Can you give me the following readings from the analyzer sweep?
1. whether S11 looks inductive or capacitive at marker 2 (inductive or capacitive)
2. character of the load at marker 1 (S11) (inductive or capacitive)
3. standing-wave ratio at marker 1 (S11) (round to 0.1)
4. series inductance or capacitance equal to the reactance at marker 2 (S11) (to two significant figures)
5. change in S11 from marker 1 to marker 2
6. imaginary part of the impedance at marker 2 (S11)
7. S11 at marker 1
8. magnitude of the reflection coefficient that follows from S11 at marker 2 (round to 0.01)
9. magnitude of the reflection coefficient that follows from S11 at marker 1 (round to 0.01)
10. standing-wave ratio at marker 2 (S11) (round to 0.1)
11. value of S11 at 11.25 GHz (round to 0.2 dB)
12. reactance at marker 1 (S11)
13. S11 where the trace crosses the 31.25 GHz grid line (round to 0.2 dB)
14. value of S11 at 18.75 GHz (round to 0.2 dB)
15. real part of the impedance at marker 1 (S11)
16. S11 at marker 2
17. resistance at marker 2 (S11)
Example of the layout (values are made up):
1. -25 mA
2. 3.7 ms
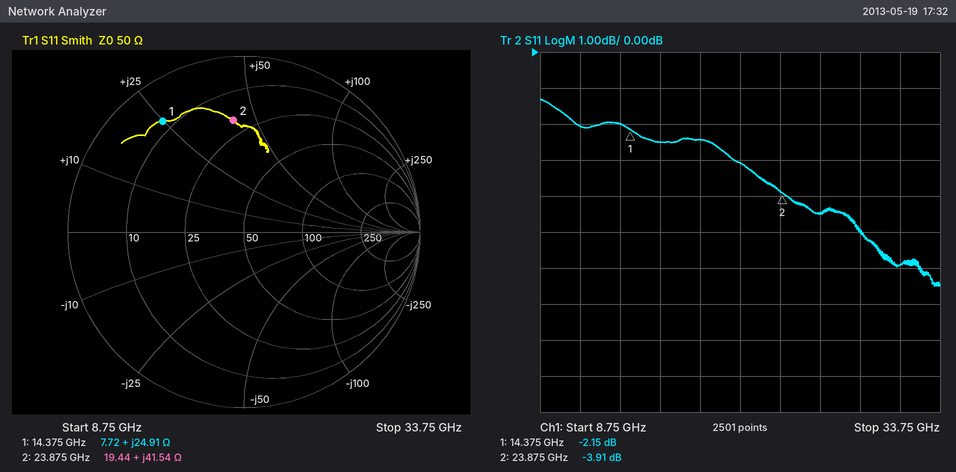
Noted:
1. inductive
2. inductive
3. 8.1
4. 280 pH
5. -1.76 dB
6. +41.54 Ω
7. -2.15 dB
8. 0.64
9. 0.78
10. 4.5
11. -2.0 dB
12. +24.91 Ω
13. -6.0 dB
14. -2.4 dB
15. 7.72 Ω
16. -3.91 dB
17. 19.44 Ω
